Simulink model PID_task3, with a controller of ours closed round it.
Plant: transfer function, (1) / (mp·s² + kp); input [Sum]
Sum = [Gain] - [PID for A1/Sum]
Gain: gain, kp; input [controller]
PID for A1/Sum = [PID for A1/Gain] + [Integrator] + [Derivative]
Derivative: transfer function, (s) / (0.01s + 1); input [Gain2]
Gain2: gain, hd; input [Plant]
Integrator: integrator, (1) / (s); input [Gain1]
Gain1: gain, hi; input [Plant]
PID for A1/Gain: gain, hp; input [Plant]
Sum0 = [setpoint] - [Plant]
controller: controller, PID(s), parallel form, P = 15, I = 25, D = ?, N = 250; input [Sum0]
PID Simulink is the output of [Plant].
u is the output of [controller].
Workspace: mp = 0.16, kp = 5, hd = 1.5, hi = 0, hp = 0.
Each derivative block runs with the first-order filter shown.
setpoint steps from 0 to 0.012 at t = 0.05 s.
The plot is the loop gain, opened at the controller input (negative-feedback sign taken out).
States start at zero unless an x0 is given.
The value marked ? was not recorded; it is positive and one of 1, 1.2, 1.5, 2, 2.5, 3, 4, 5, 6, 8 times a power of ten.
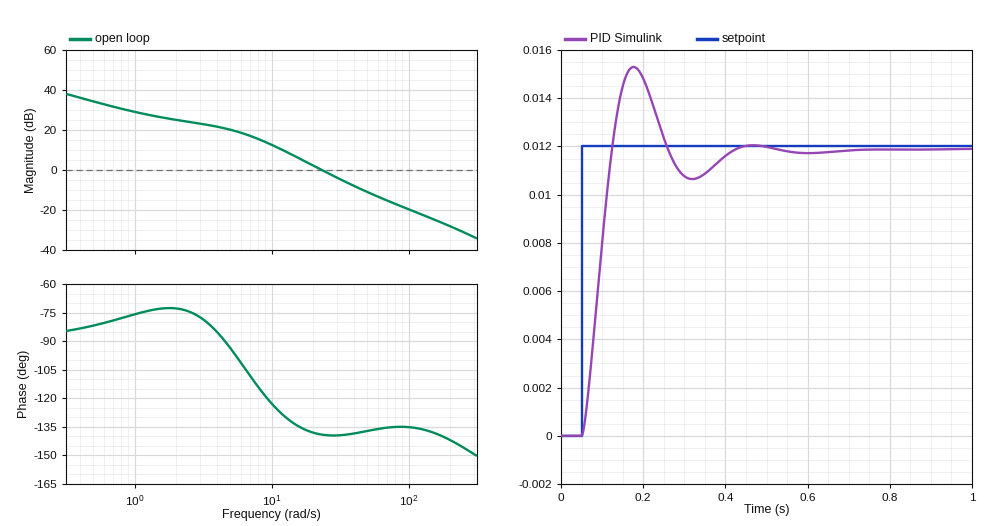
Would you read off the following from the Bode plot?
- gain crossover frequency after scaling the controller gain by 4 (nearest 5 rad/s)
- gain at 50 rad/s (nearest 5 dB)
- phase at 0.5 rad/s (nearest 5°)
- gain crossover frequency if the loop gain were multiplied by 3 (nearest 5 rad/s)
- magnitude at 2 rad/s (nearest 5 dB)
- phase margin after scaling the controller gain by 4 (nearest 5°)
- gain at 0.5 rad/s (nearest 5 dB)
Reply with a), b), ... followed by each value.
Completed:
a) 55 rad/s
b) -10 dB
c) -80°
d) 45 rad/s
e) 25 dB
f) 45°
g) 35 dB
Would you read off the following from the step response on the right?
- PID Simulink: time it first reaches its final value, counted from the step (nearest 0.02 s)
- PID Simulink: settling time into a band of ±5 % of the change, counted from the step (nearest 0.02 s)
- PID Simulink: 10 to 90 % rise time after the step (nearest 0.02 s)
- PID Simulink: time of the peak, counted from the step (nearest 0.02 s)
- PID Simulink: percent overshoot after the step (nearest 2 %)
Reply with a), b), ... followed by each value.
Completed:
a) 0.08 s
b) 0.34 s
c) 0.06 s
d) 0.12 s
e) 28 %
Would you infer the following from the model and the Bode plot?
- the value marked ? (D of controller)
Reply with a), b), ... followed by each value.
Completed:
a) 0.25
